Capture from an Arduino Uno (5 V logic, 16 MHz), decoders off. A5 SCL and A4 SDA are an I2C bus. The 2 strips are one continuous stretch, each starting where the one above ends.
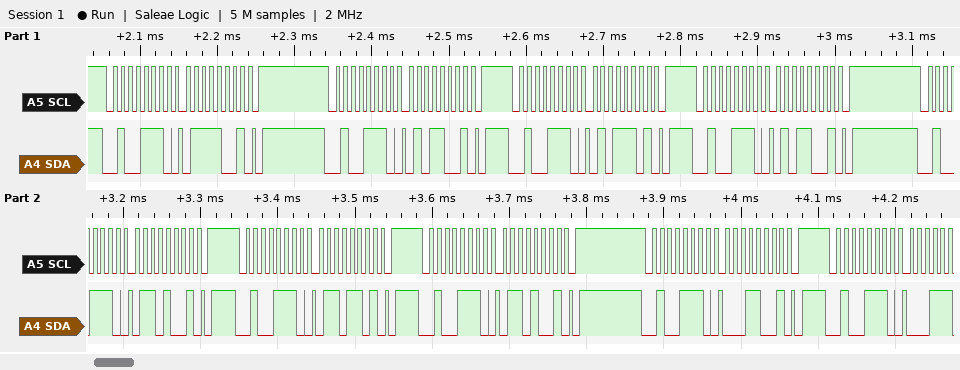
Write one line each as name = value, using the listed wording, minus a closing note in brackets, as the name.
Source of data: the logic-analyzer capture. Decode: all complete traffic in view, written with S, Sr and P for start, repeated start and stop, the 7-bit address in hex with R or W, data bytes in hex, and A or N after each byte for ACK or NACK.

all complete traffic in view, written with S, Sr and P for start, repeated start and stop, the 7-bit address in hex with R or W, data bytes in hex, and A or N after each byte for ACK or NACK = S 27W A 79 A P S 27W A 59 A P S 27W A 5D A P S 27W A 59 A P S 27W A 69 A P S 27W A 6D A P S 27W A 69 A P S 27W A 19 A P S 27W A
